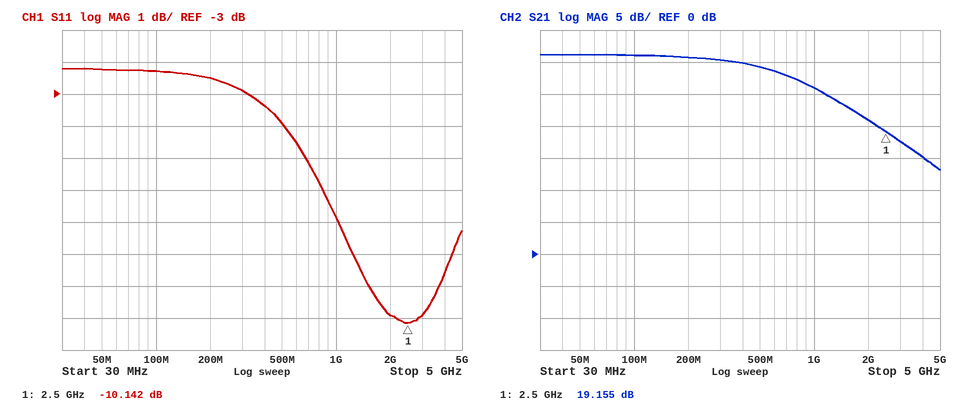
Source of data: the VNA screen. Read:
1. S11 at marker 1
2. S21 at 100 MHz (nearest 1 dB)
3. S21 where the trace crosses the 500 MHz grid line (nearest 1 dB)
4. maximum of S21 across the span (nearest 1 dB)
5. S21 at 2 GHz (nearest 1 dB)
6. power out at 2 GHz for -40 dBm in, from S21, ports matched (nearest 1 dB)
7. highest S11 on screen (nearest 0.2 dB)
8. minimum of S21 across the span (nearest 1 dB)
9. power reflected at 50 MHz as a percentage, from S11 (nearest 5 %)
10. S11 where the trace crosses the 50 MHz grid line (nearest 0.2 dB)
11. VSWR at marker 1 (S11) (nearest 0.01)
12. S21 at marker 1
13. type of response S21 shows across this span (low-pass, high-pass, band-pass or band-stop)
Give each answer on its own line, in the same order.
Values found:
-10.142 dB
31 dB
29 dB
31 dB
21 dB
-19 dBm
-2.2 dB
13 dB
60 %
-2.2 dB
1.90
19.155 dB
low-pass
